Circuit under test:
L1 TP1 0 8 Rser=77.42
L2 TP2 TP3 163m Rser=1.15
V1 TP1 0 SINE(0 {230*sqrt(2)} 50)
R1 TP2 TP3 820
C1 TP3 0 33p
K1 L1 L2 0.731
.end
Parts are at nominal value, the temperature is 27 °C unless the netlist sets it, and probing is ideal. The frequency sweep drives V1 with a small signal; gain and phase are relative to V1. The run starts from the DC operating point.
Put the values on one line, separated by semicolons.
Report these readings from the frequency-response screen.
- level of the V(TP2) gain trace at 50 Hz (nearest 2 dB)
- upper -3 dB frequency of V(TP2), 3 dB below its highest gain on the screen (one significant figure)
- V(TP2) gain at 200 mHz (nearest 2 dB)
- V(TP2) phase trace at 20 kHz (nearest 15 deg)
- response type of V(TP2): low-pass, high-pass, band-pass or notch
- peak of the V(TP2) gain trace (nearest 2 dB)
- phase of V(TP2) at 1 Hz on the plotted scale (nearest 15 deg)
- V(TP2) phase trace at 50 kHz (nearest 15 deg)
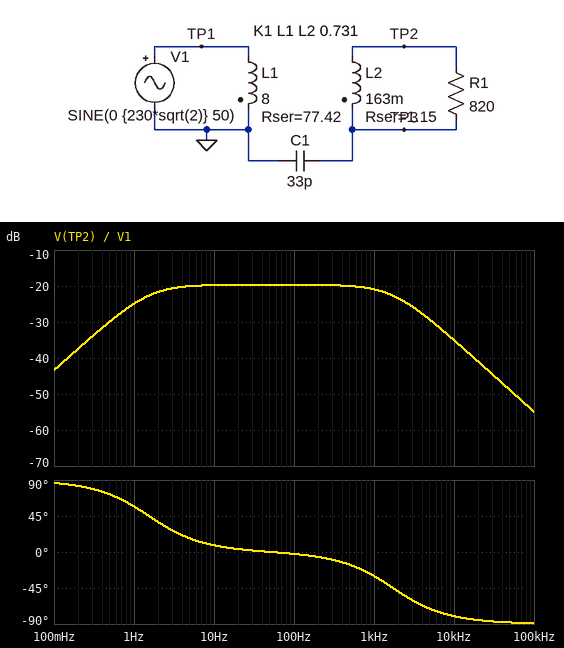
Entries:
-20 dB; 2 kHz; -38 dB; -90 deg; band-pass; -20 dB; 60 deg; -90 deg
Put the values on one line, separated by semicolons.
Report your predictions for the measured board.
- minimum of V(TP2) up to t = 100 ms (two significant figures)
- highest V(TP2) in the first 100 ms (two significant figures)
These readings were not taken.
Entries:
-35 V; 33 V
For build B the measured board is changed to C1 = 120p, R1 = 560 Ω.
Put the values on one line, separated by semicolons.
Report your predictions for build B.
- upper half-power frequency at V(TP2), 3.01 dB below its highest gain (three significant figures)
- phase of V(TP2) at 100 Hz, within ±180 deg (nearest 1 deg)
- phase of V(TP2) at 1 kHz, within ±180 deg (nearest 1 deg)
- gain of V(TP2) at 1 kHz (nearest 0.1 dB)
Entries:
1.18 kHz; -4 deg; -40 deg; -22.0 dB
